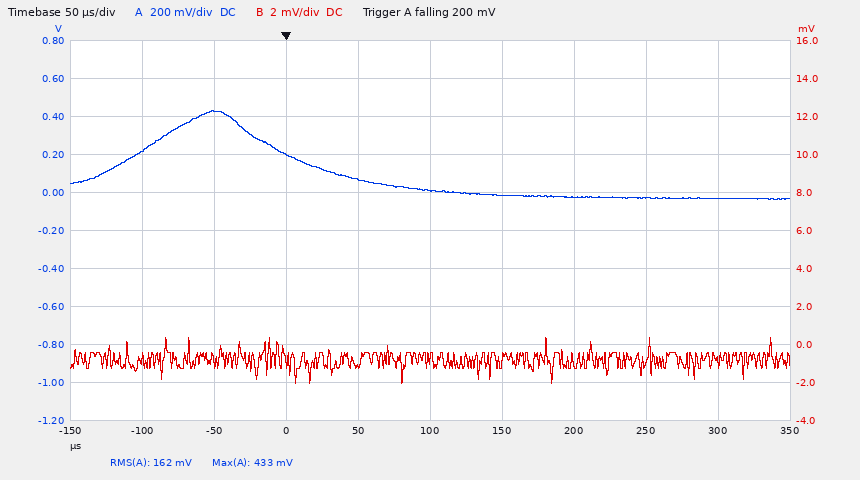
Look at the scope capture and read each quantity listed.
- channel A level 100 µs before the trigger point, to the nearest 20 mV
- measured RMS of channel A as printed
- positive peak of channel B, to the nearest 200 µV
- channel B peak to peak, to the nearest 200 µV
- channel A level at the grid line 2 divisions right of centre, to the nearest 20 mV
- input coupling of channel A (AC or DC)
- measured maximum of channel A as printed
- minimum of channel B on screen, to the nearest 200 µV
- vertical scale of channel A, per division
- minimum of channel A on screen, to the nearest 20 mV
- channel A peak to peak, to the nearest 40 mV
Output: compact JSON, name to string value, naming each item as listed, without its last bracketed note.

{"channel A level 100 µs before the trigger point, to the nearest 20 mV": "220 mV", "measured RMS of channel A as printed": "162 mV", "positive peak of channel B, to the nearest 200 µV": "400 µV", "channel B peak to peak, to the nearest 200 µV": "2.4 mV", "channel A level at the grid line 2 divisions right of centre, to the nearest 20 mV": "-20 mV", "input coupling of channel A": "DC", "measured maximum of channel A as printed": "433 mV", "minimum of channel B on screen, to the nearest 200 µV": "-2.0 mV", "vertical scale of channel A, per division": "200 mV", "minimum of channel A on screen, to the nearest 20 mV": "-40 mV", "channel A peak to peak, to the nearest 40 mV": "480 mV"}
